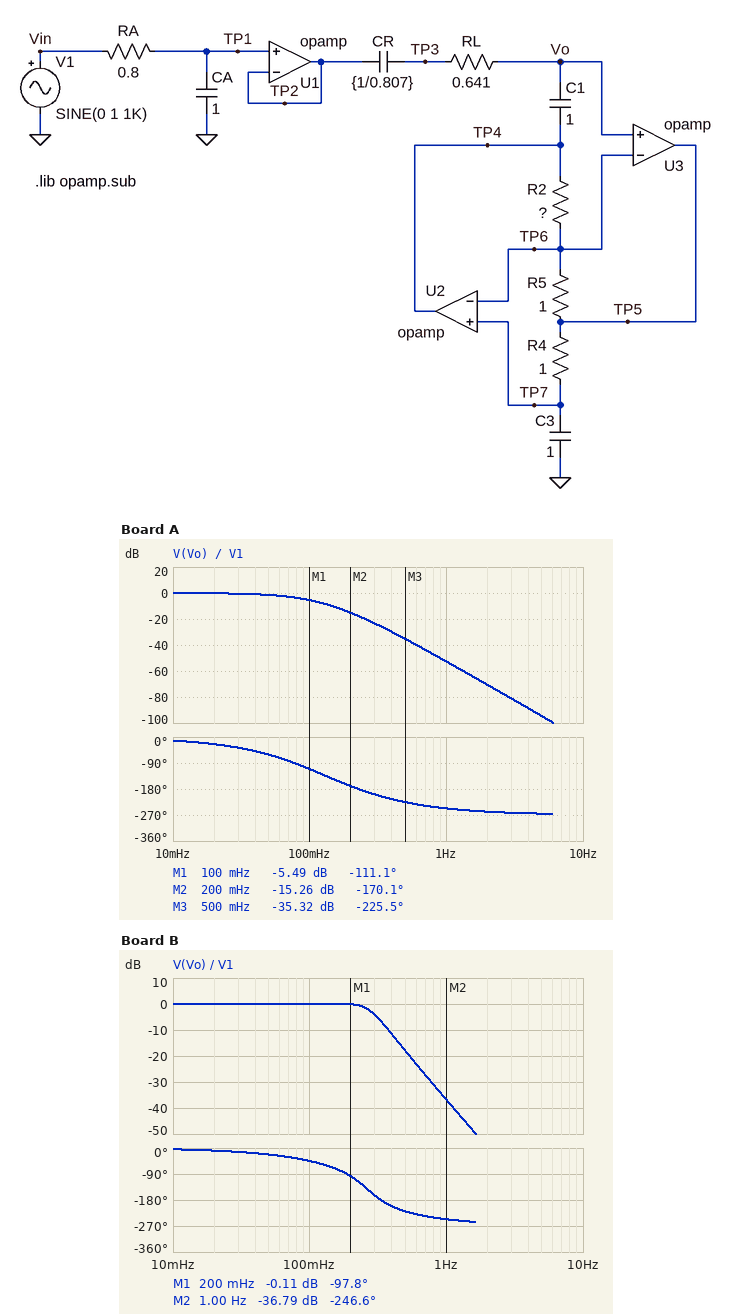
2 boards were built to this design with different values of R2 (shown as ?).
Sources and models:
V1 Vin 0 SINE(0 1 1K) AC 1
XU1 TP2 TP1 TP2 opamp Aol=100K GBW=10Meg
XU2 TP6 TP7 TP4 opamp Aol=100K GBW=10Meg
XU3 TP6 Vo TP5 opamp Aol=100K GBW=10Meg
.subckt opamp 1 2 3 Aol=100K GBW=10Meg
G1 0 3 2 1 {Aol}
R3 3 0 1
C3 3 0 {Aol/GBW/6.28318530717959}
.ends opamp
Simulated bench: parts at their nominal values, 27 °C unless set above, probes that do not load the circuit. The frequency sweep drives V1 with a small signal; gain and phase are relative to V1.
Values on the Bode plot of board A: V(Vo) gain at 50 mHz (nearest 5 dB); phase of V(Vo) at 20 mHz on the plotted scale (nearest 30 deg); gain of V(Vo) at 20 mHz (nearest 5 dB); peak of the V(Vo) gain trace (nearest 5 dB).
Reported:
0 dB
-30 deg
0 dB
0 dB
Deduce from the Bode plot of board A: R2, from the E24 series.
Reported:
3.3 Ω
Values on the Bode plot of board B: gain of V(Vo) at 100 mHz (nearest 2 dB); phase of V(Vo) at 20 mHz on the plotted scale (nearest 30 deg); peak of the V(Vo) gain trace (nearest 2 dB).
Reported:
0 dB
0 deg
0 dB
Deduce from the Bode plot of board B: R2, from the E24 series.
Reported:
0.56 Ω
